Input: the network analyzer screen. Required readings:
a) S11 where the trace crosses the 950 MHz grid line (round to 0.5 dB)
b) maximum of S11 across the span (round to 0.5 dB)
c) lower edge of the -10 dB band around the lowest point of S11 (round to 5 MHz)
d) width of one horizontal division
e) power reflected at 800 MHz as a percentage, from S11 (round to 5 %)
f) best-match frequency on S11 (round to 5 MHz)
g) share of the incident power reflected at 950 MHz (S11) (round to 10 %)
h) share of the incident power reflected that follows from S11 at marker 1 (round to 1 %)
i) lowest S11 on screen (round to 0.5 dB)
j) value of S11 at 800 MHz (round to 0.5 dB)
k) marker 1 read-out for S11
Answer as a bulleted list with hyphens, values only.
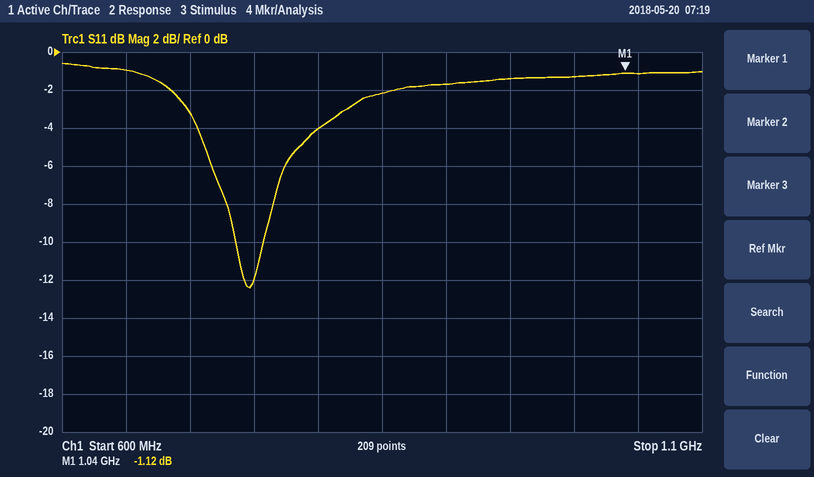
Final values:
- -1.5 dB
- -0.5 dB
- 735 MHz
- 50 MHz
- 40 %
- 745 MHz
- 70 %
- 77 %
- -12.5 dB
- -4.0 dB
- -1.12 dB
